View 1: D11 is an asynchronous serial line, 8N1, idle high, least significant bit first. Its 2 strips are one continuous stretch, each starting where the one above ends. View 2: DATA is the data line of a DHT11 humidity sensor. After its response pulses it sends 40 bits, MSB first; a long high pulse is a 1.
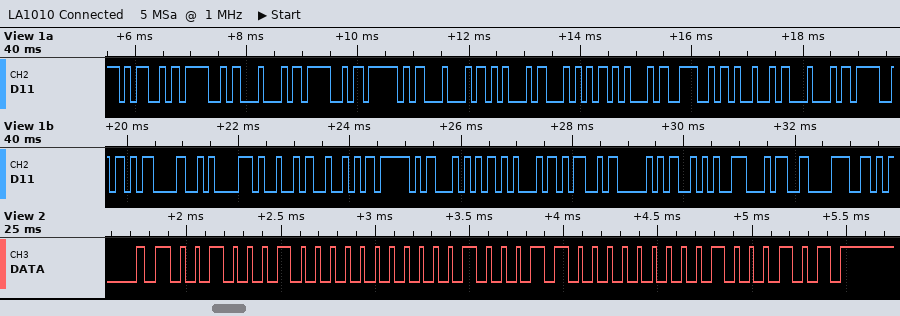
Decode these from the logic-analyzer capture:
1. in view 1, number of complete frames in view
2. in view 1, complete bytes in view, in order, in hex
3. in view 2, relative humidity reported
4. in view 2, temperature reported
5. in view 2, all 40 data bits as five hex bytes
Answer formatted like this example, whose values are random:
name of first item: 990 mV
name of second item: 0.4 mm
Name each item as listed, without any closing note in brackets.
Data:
in view 1, number of complete frames in view: 25
in view 1, complete bytes in view, in order, in hex: 4D 4F 44 4F 5F 44 45 54 45 4E 49 44 4F 0D 0A 49 52 5F 54 45 4D 50 2A 34 38
in view 2, relative humidity reported: 34 %
in view 2, temperature reported: 35.0 °C
in view 2, all 40 data bits as five hex bytes: 22 00 23 00 45
